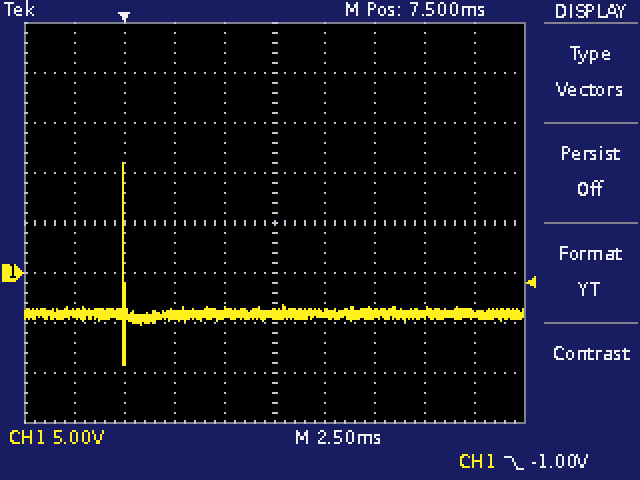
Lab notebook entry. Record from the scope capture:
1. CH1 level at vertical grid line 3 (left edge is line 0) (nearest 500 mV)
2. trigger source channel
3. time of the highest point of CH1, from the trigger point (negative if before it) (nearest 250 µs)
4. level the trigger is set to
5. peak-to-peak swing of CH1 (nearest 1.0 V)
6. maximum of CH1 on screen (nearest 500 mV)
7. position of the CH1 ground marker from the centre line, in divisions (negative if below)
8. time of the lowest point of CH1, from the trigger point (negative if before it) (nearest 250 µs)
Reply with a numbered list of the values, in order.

1. -4.0 V
2. CH1
3. 0.00 ms
4. -1.00 V
5. 20.0 V
6. 11.0 V
7. -1.0 div
8. 0.00 ms
